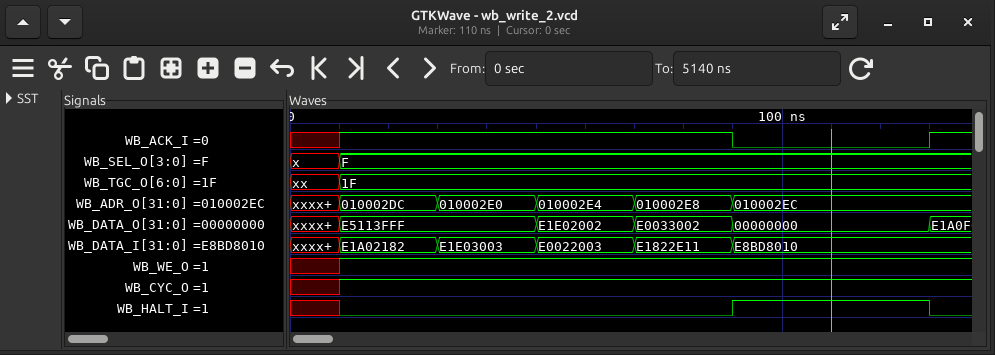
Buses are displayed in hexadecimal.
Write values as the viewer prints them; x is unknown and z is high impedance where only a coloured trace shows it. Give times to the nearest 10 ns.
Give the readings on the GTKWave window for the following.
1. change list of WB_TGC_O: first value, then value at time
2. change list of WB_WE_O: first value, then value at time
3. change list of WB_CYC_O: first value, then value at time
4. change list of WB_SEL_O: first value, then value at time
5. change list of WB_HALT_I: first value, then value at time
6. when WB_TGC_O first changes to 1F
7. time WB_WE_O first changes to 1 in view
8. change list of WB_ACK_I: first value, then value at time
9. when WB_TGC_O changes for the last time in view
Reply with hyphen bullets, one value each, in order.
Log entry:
- xx, 1F at 10 ns
- x, 1 at 10 ns
- x, 1 at 10 ns
- x, F at 10 ns
- x, 0 at 10 ns, 1 at 90 ns, 0 at 130 ns
- 10 ns
- 10 ns
- x, 1 at 10 ns, 0 at 90 ns, 1 at 130 ns
- 10 ns
